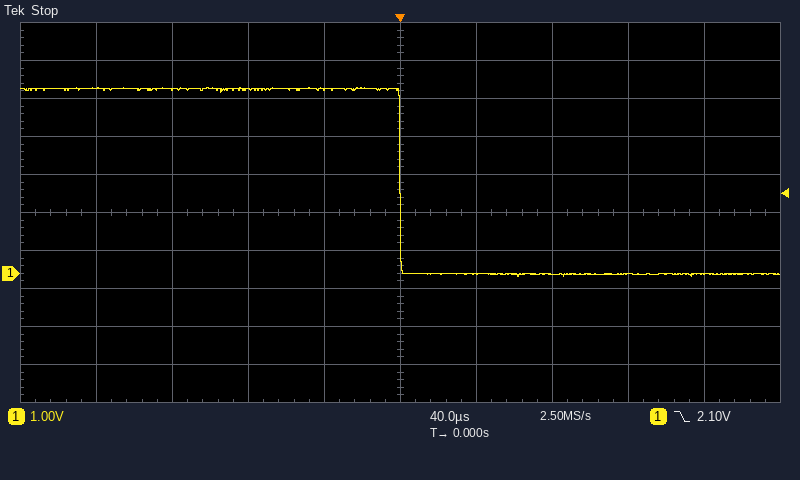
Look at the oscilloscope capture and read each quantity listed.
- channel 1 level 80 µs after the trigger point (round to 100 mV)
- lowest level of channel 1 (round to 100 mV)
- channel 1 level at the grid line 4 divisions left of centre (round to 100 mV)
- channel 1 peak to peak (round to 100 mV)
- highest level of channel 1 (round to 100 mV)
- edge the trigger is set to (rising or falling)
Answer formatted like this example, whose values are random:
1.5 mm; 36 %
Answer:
0.0 V; -100 mV; 4.9 V; 5.0 V; 4.9 V; falling
